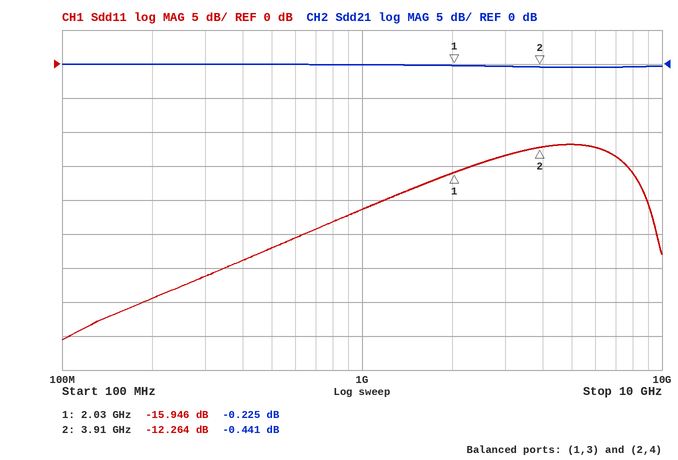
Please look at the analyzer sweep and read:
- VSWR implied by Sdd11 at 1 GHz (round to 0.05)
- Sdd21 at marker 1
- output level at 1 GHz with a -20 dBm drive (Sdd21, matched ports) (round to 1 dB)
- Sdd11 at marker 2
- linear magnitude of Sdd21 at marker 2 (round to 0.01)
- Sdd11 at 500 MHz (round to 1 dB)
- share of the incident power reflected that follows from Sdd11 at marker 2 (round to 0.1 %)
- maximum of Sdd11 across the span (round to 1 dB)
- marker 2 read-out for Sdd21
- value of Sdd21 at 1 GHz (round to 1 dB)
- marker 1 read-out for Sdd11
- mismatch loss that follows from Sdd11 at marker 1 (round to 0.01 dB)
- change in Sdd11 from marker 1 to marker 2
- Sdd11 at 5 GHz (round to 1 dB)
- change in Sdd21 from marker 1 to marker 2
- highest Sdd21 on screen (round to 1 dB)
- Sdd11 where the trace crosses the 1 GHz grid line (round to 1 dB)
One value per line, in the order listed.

1.20
-0.225 dB
-20 dBm
-12.264 dB
0.95
-27 dB
5.9 %
-12 dB
-0.441 dB
0 dB
-15.946 dB
0.11 dB
3.682 dB
-12 dB
-0.216 dB
0 dB
-21 dB
